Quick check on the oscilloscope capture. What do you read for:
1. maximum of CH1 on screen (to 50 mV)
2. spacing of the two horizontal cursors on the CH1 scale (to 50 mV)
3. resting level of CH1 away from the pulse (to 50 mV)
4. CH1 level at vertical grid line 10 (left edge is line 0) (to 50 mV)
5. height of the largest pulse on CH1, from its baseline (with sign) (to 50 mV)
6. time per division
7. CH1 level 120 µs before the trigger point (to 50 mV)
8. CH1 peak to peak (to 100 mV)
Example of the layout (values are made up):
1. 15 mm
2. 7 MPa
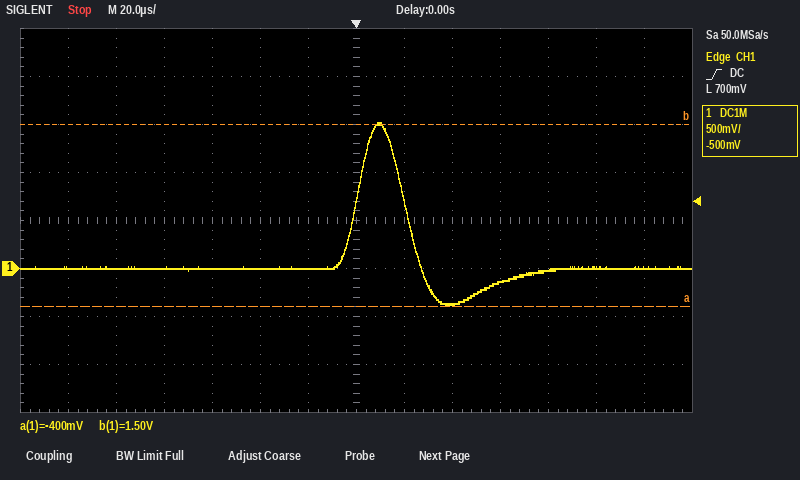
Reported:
1. 1.50 V
2. 1.90 V
3. 0 mV
4. -150 mV
5. +1.50 V
6. 20 µs
7. 0 mV
8. 1.90 V
